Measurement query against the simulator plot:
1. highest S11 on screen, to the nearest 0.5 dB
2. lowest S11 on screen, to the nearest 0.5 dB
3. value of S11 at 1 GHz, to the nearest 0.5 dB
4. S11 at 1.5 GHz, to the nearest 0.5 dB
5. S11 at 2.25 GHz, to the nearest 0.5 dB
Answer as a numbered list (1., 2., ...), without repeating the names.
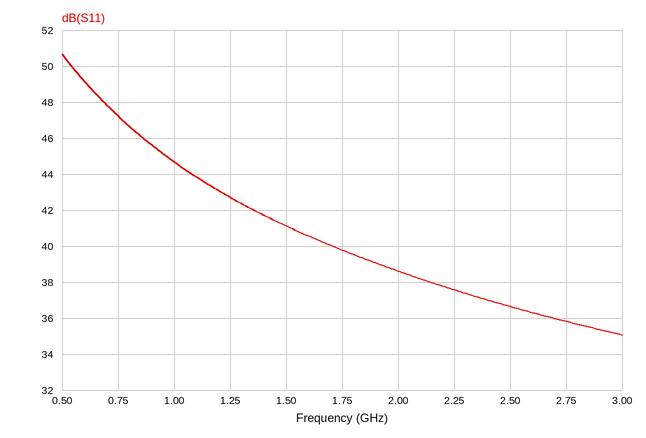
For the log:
1. 50.5 dB
2. 35.0 dB
3. 44.5 dB
4. 41.0 dB
5. 37.5 dB
